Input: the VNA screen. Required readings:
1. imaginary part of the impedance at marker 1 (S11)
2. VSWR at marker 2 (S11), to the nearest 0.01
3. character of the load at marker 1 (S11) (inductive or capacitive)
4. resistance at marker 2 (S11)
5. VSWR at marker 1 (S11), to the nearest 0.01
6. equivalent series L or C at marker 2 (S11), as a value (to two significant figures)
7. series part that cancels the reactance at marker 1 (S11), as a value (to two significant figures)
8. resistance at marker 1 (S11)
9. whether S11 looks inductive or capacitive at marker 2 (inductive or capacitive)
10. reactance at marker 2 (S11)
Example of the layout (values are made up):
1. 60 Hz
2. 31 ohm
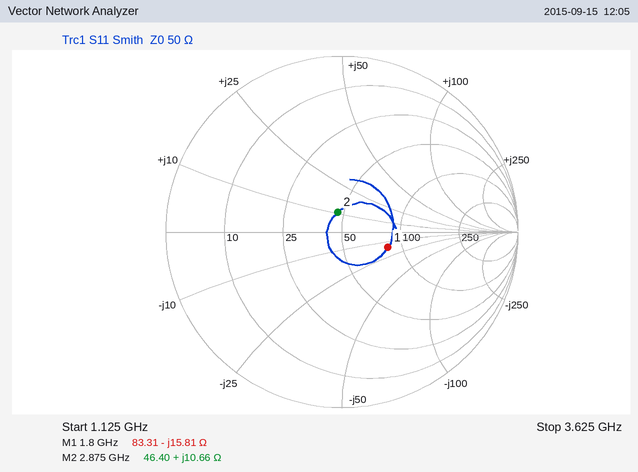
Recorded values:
1. -15.81 Ω
2. 1.26
3. capacitive
4. 46.40 Ω
5. 1.76
6. 590 pH
7. 1.4 nH
8. 83.31 Ω
9. inductive
10. +10.66 Ω
